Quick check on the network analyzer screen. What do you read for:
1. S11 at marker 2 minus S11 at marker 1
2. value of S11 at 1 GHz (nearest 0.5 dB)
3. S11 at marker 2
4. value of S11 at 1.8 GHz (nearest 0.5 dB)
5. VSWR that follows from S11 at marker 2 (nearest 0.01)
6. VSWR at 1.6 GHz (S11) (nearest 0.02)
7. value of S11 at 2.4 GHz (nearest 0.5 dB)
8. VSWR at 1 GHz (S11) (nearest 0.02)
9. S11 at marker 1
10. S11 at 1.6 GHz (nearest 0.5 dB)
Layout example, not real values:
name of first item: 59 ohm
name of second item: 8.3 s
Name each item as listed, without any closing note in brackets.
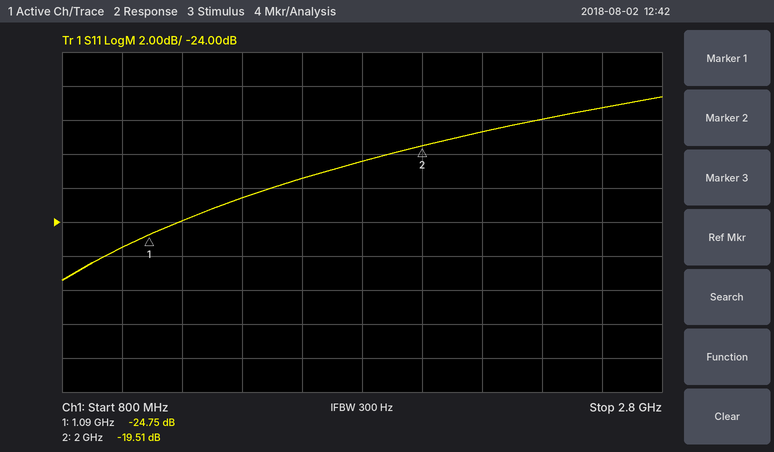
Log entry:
S11 at marker 2 minus S11 at marker 1: 5.24 dB
value of S11 at 1 GHz: -25.5 dB
S11 at marker 2: -19.51 dB
value of S11 at 1.8 GHz: -20.5 dB
VSWR that follows from S11 at marker 2: 1.24
VSWR at 1.6 GHz (S11): 1.18
value of S11 at 2.4 GHz: -18.0 dB
VSWR at 1 GHz (S11): 1.12
S11 at marker 1: -24.75 dB
S11 at 1.6 GHz: -21.5 dB
